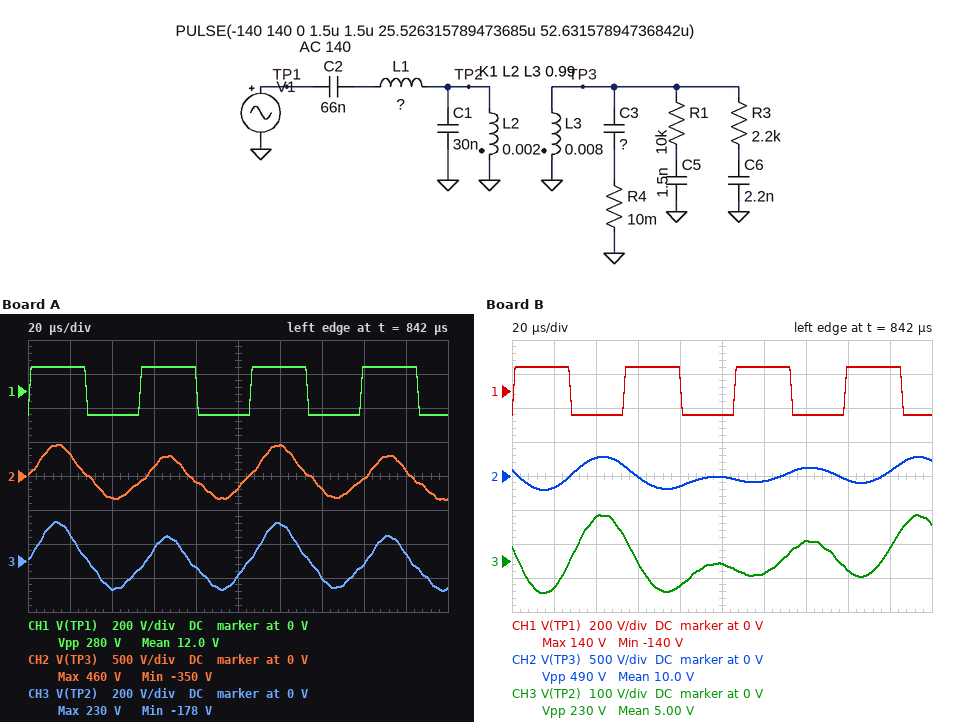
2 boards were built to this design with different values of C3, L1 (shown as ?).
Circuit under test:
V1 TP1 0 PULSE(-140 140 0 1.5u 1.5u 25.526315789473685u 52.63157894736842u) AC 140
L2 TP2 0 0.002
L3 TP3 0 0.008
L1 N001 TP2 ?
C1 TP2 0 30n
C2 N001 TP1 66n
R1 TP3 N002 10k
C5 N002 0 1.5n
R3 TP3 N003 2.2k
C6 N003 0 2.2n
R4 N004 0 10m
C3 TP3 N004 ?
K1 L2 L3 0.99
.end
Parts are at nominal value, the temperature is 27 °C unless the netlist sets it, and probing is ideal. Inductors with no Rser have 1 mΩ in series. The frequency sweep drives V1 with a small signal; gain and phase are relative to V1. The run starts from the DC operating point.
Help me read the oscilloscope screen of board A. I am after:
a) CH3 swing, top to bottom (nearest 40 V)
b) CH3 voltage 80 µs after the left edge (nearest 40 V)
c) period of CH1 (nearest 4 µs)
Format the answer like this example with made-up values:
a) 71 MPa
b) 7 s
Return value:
a) 400 V
b) -40 V
c) 52 µs
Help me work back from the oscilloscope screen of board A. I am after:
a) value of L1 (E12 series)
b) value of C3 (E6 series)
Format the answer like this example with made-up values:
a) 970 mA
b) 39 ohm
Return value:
a) 820 µH
b) 6.8 nF
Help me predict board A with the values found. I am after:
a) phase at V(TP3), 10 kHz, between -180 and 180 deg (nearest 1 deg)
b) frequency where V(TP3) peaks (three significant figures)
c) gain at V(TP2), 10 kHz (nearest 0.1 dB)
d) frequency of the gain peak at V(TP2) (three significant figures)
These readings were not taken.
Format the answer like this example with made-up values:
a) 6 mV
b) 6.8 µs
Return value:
a) 12 deg
b) 9.22 kHz
c) 10.3 dB
d) 9.22 kHz
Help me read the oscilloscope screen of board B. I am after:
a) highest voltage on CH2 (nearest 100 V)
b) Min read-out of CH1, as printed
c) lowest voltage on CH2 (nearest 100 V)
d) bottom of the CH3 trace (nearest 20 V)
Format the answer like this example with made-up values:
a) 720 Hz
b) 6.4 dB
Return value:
a) 300 V
b) -140 V
c) -200 V
d) -100 V
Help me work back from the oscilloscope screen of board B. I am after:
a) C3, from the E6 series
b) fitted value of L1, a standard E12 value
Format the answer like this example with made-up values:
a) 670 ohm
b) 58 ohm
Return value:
a) 33 nF
b) 2.7 mH
